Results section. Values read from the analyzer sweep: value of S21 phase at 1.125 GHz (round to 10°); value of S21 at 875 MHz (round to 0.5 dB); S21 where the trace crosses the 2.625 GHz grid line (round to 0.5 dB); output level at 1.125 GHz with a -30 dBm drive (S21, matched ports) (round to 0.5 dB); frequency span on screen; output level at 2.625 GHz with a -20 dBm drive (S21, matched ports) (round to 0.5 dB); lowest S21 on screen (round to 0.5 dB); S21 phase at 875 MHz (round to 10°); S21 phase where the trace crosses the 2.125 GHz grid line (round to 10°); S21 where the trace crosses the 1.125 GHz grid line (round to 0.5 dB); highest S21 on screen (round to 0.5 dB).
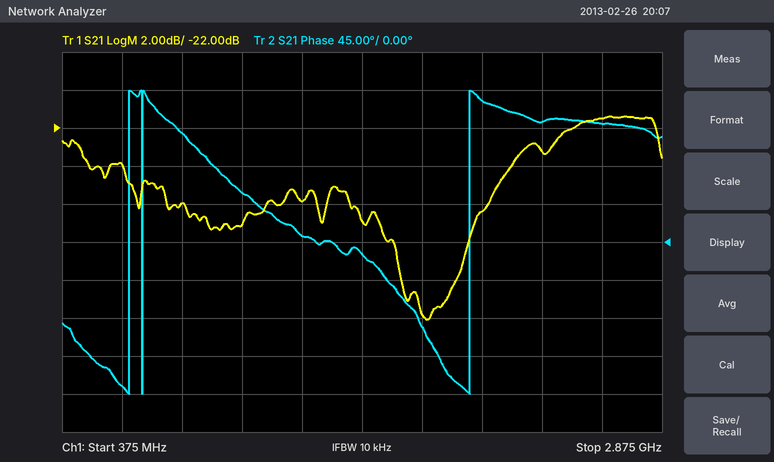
60°
-26.0 dB
-21.5 dB
-57.0 dBm
2.5 GHz
-41.5 dBm
-32.0 dB
130°
170°
-27.0 dB
-21.5 dB
